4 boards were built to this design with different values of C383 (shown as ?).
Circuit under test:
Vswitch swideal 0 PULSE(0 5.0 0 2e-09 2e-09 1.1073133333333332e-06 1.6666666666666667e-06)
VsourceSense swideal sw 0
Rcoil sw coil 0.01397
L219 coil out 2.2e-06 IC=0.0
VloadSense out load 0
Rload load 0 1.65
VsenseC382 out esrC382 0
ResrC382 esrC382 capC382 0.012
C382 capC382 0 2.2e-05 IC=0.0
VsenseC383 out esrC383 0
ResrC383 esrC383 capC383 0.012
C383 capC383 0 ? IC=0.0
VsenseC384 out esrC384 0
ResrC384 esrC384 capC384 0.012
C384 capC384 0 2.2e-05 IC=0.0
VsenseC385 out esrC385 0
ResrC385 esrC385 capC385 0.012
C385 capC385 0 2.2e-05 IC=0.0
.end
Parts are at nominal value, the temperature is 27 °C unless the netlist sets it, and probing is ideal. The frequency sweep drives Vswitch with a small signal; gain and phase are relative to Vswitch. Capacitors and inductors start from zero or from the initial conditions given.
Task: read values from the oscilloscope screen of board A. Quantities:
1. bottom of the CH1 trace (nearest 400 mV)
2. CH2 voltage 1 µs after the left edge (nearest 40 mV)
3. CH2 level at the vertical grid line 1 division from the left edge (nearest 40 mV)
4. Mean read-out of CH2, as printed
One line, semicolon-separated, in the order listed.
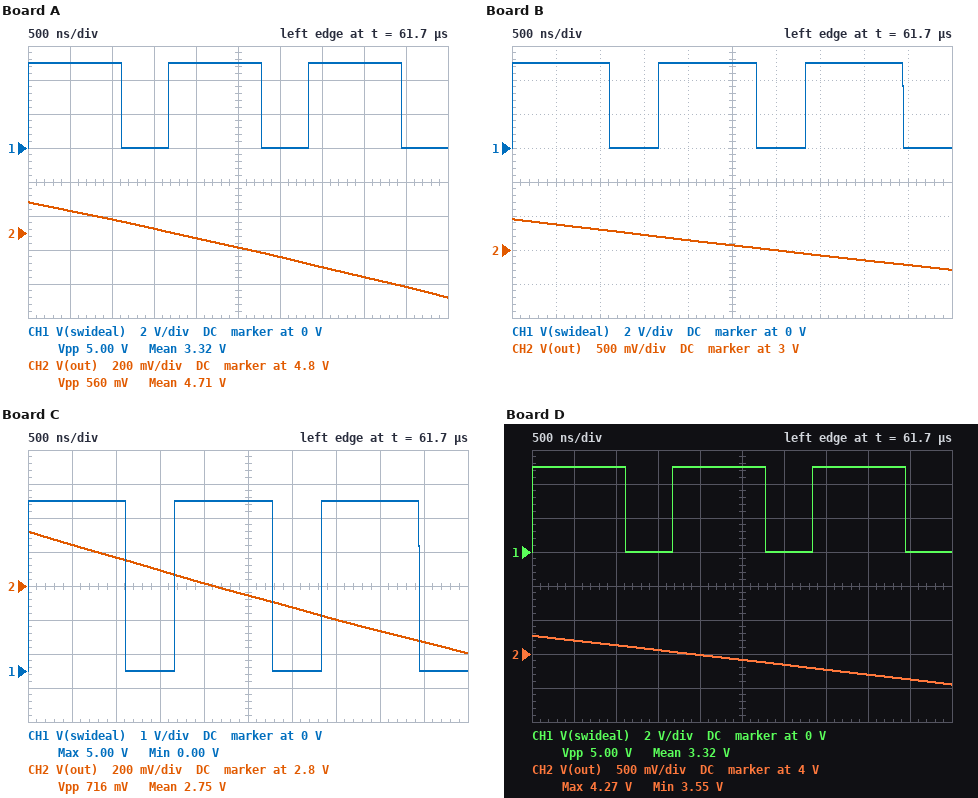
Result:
0 V; 4.88 V; 4.92 V; 4.71 V
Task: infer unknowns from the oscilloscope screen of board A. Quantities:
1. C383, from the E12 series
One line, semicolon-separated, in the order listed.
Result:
47 µF
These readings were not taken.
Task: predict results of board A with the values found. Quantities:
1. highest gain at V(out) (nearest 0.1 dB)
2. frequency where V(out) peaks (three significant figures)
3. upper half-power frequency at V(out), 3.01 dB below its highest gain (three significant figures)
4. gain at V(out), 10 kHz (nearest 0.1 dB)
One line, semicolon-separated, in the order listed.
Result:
13.6 dB; 10.0 kHz; 11.0 kHz; 13.6 dB
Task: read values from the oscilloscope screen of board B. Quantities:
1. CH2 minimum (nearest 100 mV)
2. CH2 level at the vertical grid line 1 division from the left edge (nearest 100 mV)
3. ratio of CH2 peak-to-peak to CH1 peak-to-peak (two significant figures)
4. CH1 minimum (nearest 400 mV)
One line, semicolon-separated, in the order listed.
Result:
2.7 V; 3.4 V; 0.15; 0 V
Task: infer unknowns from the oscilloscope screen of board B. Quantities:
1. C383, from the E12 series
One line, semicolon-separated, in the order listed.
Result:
12 µF
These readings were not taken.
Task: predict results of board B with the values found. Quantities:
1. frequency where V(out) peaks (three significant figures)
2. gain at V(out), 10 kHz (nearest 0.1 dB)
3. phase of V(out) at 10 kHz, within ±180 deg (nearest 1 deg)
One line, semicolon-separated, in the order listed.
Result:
12.1 kHz; 8.6 dB; -26 deg
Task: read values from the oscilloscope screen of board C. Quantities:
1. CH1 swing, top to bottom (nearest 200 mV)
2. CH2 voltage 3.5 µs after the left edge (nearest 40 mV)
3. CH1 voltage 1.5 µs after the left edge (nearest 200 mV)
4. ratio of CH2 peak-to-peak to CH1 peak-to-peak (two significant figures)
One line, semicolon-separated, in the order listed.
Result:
5.0 V; 2.60 V; 0 V; 0.14
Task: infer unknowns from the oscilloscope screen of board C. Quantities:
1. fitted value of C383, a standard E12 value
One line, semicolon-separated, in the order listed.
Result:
6.8 µF
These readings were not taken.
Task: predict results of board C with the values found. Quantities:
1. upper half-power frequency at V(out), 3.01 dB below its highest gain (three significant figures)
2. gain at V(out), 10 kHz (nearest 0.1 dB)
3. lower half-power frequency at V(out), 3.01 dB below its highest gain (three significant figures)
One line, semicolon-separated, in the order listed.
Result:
13.7 kHz; 7.8 dB; 11.1 kHz
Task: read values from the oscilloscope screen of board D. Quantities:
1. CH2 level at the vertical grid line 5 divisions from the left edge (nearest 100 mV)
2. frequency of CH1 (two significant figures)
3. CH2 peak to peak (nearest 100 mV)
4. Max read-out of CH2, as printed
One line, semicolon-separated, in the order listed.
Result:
3.9 V; 600 kHz; 700 mV; 4.27 V
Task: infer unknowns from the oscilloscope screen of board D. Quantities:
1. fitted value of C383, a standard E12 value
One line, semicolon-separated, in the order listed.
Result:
27 µF
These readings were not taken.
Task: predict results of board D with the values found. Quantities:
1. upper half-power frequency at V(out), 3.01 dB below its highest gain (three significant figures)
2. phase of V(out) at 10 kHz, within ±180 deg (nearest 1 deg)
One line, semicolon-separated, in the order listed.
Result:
12.1 kHz; -42 deg
